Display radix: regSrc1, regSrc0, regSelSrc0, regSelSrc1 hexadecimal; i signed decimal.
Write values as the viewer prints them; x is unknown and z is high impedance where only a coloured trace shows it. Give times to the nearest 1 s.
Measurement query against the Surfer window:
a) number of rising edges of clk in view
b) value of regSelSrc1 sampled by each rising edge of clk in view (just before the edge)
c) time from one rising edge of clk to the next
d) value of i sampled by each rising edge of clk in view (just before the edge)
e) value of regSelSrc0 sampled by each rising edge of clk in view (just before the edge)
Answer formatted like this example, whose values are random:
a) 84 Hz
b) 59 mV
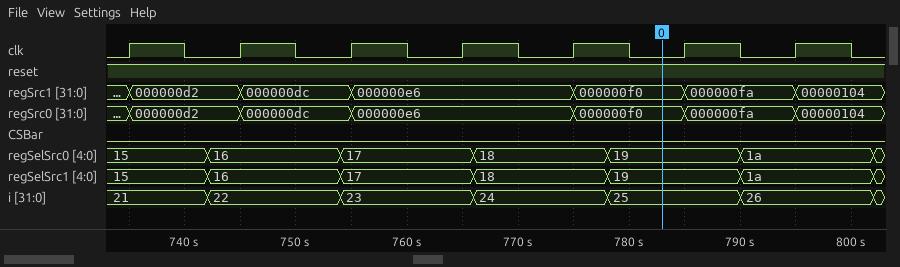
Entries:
a) 7
b) 15, 16, 17, 17, 18, 19, 1a
c) 10 s
d) 21, 22, 23, 23, 24, 25, 26
e) 15, 16, 17, 17, 18, 19, 1a
